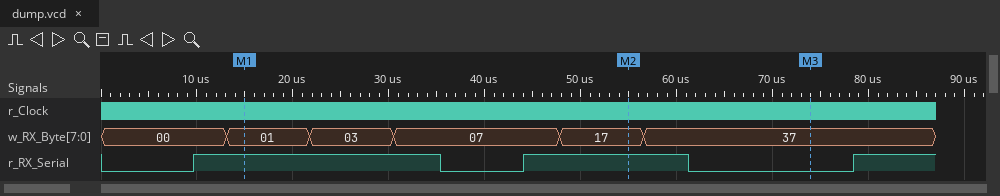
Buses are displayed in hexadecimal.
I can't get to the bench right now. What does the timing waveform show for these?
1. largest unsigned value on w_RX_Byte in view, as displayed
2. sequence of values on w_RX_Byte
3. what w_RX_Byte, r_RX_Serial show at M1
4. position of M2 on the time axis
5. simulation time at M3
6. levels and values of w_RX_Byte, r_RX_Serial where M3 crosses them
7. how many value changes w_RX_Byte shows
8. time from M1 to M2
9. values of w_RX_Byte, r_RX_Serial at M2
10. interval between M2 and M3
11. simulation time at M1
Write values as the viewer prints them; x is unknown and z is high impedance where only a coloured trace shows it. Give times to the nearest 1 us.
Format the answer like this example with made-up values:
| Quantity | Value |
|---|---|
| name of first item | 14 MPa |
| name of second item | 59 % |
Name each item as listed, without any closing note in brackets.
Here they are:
| Quantity | Value |
|---|---|
| largest unsigned value on w_RX_Byte in view, as displayed | 37 |
| sequence of values on w_RX_Byte | 00, 01, 03, 07, 17, 37 |
| what w_RX_Byte, r_RX_Serial show at M1 | w_RX_Byte=01, r_RX_Serial=1 |
| position of M2 on the time axis | 55 us |
| simulation time at M3 | 74 us |
| levels and values of w_RX_Byte, r_RX_Serial where M3 crosses them | w_RX_Byte=37, r_RX_Serial=0 |
| how many value changes w_RX_Byte shows | 5 |
| time from M1 to M2 | 40 us |
| values of w_RX_Byte, r_RX_Serial at M2 | w_RX_Byte=17, r_RX_Serial=1 |
| interval between M2 and M3 | 19 us |
| simulation time at M1 | 15 us |
